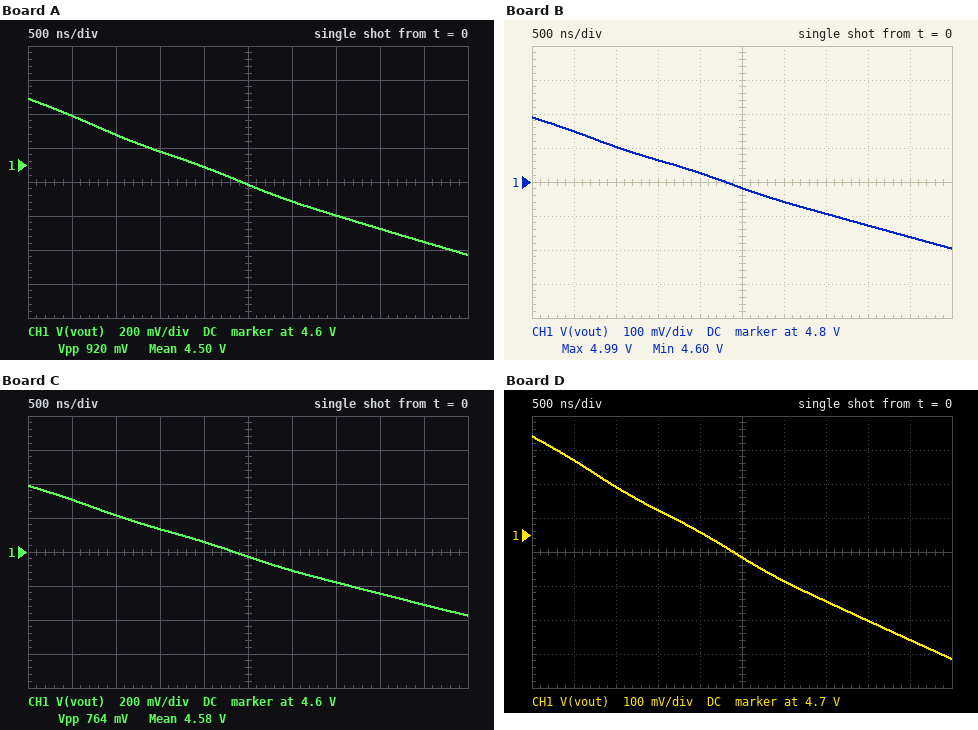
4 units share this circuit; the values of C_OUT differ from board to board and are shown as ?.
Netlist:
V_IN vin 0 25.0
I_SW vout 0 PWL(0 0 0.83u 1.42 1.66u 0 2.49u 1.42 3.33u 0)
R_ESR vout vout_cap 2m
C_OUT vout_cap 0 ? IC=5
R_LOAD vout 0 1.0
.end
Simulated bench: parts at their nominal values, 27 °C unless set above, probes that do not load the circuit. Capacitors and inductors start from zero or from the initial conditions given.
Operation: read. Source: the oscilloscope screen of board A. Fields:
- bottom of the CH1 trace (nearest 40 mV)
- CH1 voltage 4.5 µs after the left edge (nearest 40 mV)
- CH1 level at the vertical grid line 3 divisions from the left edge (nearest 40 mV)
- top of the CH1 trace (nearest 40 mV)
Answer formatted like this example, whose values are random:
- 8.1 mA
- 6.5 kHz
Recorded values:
- 4.08 V
- 4.16 V
- 4.68 V
- 5.00 V
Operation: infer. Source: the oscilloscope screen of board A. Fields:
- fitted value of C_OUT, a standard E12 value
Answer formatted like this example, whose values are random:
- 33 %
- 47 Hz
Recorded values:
- 27 µF
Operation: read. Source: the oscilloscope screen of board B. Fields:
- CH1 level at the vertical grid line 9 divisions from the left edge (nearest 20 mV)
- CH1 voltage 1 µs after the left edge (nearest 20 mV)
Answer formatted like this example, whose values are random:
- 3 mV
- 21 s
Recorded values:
- 4.64 V
- 4.90 V
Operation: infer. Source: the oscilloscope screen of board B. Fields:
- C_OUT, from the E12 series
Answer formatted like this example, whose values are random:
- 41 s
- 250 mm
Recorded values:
- 68 µF
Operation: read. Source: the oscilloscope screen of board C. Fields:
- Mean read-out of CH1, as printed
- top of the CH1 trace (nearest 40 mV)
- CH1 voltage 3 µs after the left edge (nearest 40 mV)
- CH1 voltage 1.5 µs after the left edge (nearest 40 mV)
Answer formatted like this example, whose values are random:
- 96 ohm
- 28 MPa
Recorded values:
- 4.58 V
- 5.00 V
- 4.48 V
- 4.72 V
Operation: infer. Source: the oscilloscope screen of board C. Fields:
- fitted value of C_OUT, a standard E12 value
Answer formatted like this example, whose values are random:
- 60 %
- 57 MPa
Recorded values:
- 33 µF
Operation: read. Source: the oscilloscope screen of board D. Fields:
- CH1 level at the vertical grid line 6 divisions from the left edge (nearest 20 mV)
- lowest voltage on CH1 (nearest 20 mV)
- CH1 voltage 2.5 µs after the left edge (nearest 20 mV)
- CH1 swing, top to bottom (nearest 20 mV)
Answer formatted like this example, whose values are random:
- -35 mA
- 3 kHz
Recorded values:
- 4.56 V
- 4.34 V
- 4.64 V
- 660 mV
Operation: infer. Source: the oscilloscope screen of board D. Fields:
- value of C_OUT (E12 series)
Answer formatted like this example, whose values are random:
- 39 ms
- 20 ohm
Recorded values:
- 39 µF
